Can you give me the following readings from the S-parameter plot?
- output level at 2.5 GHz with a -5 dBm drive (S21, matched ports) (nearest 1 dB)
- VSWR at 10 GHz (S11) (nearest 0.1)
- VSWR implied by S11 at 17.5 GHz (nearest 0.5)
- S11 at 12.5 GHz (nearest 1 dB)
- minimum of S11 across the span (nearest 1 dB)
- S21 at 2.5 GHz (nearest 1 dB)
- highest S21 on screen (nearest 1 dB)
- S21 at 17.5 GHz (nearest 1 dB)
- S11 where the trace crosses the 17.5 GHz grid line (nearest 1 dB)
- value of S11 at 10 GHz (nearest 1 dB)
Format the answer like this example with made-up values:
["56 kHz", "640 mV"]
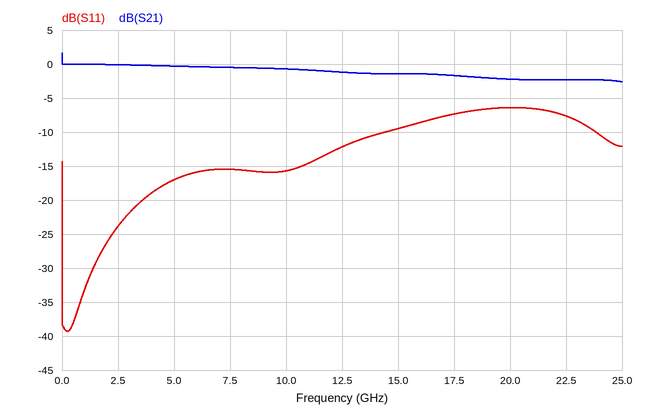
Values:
["-5 dBm", "1.4", "2.5", "-12 dB", "-39 dB", "0 dB", "2 dB", "-2 dB", "-7 dB", "-16 dB"]
